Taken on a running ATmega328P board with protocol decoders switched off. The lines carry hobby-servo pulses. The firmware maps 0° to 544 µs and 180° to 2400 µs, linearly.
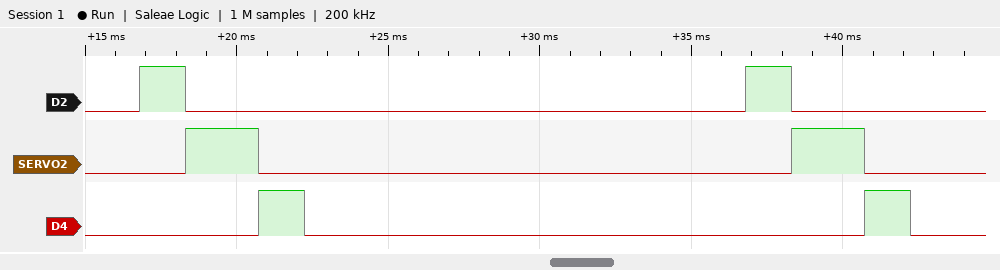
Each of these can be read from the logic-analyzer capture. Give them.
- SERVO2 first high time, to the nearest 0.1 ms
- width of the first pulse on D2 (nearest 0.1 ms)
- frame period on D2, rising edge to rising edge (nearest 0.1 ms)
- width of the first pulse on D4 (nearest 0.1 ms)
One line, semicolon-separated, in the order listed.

2.4 ms; 1.5 ms; 20.0 ms; 1.5 ms
